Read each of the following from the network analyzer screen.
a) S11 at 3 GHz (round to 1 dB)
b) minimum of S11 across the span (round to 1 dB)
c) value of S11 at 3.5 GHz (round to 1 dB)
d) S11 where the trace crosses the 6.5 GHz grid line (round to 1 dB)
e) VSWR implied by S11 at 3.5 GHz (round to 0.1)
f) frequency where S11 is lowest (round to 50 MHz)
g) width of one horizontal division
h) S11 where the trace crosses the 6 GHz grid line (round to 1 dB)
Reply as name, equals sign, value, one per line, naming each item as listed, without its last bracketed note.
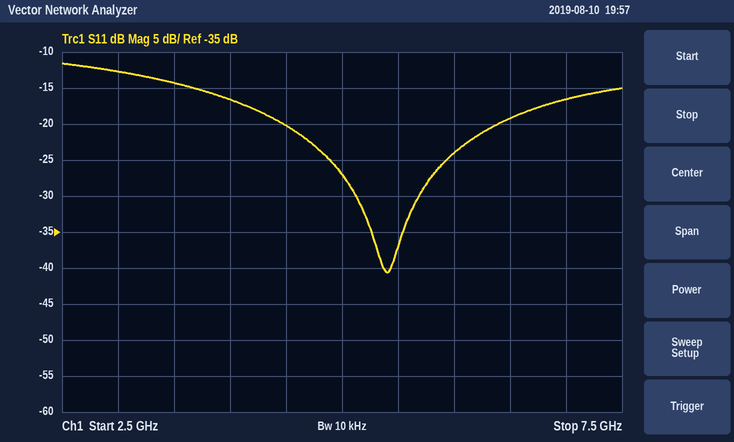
S11 at 3 GHz = -13 dB
minimum of S11 across the span = -41 dB
value of S11 at 3.5 GHz = -14 dB
S11 where the trace crosses the 6.5 GHz grid line = -19 dB
VSWR implied by S11 at 3.5 GHz = 1.5
frequency where S11 is lowest = 5.40 GHz
width of one horizontal division = 500 MHz
S11 where the trace crosses the 6 GHz grid line = -24 dB
